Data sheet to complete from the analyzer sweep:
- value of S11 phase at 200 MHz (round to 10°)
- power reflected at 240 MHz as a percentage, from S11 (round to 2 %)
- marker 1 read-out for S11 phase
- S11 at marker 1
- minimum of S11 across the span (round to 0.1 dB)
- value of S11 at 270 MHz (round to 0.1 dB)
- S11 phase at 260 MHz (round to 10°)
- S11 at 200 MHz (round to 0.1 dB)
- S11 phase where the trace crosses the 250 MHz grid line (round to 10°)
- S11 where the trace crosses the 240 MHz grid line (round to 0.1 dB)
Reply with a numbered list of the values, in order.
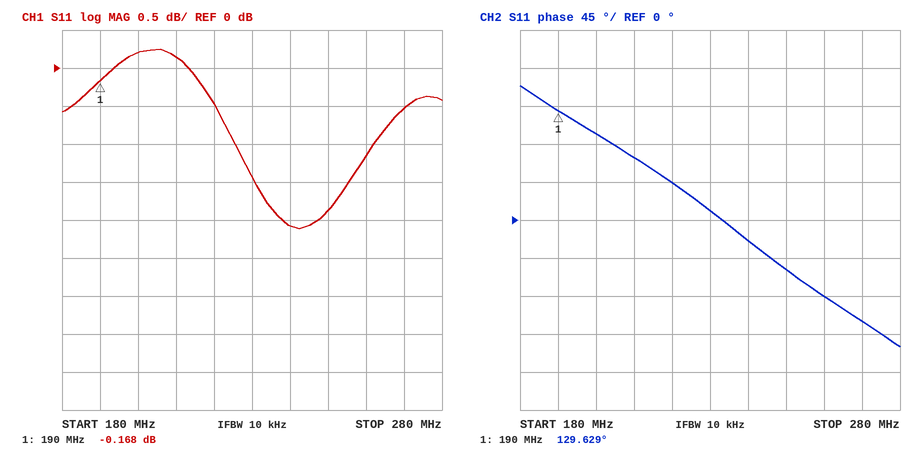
1. 100°
2. 62 %
3. 129.629°
4. -0.168 dB
5. -2.1 dB
6. -0.5 dB
7. -90°
8. 0.2 dB
9. -60°
10. -2.1 dB
